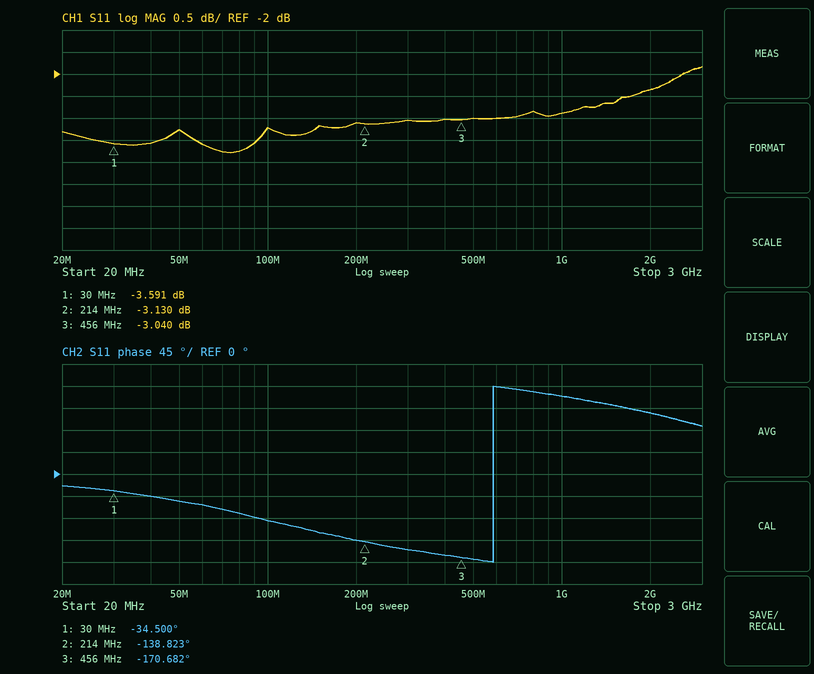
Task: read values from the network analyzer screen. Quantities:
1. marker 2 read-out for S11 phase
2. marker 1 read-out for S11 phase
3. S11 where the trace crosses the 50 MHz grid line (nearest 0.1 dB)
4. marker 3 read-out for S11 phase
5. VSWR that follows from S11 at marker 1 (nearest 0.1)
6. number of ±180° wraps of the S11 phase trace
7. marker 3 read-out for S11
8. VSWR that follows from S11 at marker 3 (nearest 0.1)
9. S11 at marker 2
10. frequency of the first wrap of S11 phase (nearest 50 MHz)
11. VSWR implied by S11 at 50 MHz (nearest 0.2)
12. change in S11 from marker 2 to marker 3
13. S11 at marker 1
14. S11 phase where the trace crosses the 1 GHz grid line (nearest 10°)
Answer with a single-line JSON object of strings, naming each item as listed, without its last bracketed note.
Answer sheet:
{"marker 2 read-out for S11 phase": "-138.823°", "marker 1 read-out for S11 phase": "-34.500°", "S11 where the trace crosses the 50 MHz grid line": "-3.3 dB", "marker 3 read-out for S11 phase": "-170.682°", "VSWR that follows from S11 at marker 1": "4.9", "number of ±180° wraps of the S11 phase trace": "1", "marker 3 read-out for S11": "-3.040 dB", "VSWR that follows from S11 at marker 3": "5.8", "S11 at marker 2": "-3.130 dB", "frequency of the first wrap of S11 phase": "600 MHz", "VSWR implied by S11 at 50 MHz": "5.4", "change in S11 from marker 2 to marker 3": "0.090 dB", "S11 at marker 1": "-3.591 dB", "S11 phase where the trace crosses the 1 GHz grid line": "160°"}
